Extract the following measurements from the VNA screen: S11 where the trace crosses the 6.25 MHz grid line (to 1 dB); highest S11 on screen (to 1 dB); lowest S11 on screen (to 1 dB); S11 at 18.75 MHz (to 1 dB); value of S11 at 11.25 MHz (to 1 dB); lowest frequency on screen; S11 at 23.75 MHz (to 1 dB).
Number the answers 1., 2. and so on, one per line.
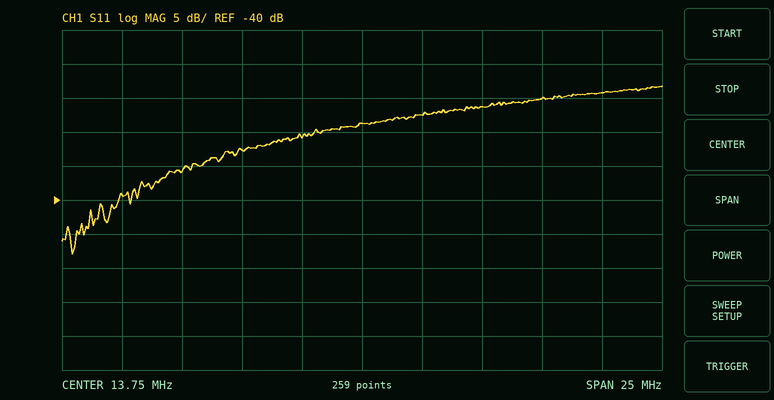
1. -36 dB
2. -23 dB
3. -48 dB
4. -26 dB
5. -31 dB
6. 1.25 MHz
7. -24 dB
